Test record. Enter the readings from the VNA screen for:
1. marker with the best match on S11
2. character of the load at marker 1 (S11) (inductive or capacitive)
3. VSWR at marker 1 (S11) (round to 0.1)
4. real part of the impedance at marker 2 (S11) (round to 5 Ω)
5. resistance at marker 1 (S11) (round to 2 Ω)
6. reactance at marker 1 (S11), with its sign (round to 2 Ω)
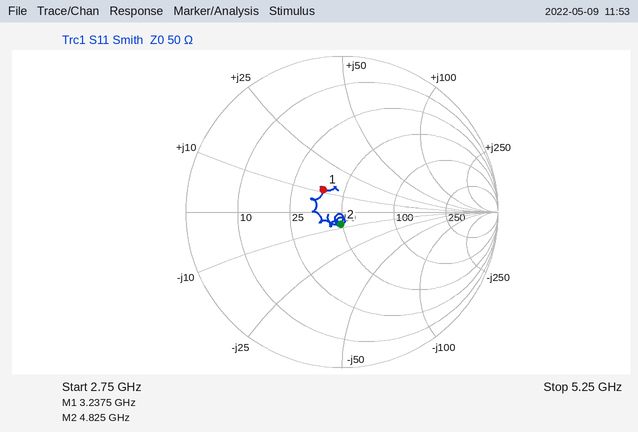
marker 2
inductive
1.5
50 Ω
38 Ω
+12 Ω
